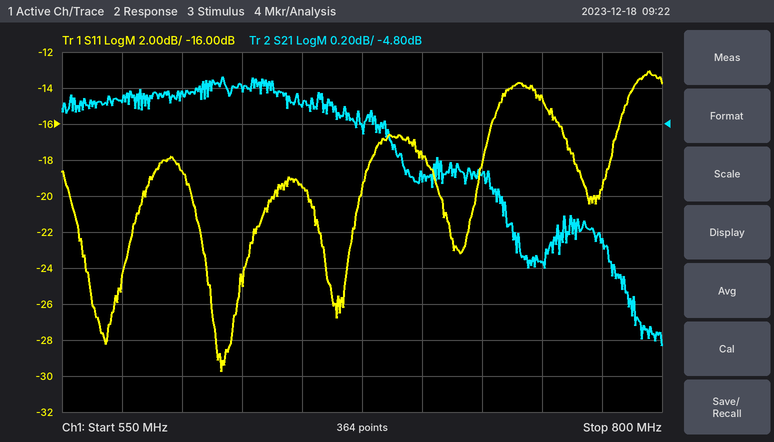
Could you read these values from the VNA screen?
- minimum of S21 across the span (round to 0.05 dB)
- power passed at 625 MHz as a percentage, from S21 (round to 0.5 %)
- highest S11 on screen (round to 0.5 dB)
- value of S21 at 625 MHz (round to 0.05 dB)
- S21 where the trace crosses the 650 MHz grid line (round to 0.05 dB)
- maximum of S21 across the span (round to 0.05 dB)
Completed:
-6.05 dB
34.5 %
-13.0 dB
-4.60 dB
-4.70 dB
-4.55 dB
